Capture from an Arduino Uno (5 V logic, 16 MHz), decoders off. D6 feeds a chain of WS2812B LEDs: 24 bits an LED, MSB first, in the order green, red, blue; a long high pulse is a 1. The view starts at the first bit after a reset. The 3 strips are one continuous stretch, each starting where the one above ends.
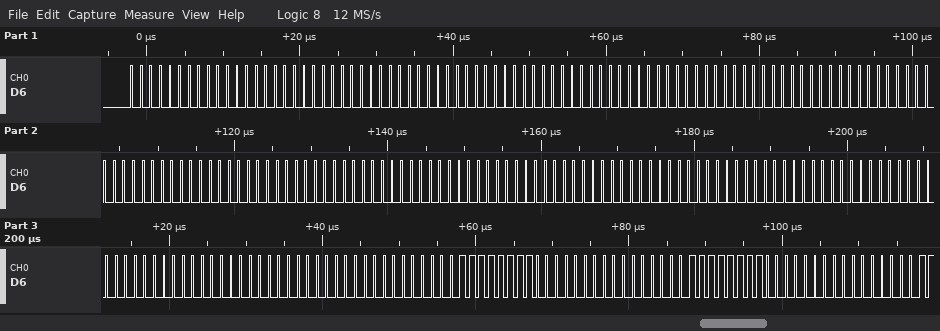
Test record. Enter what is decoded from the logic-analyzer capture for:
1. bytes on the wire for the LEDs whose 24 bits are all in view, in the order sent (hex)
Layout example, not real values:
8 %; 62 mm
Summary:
00 00 00 00 00 00 00 00 00 00 00 00 00 00 00 00 00 00 00 00 00 00 00 00 00 00 FF 00 00 FF
